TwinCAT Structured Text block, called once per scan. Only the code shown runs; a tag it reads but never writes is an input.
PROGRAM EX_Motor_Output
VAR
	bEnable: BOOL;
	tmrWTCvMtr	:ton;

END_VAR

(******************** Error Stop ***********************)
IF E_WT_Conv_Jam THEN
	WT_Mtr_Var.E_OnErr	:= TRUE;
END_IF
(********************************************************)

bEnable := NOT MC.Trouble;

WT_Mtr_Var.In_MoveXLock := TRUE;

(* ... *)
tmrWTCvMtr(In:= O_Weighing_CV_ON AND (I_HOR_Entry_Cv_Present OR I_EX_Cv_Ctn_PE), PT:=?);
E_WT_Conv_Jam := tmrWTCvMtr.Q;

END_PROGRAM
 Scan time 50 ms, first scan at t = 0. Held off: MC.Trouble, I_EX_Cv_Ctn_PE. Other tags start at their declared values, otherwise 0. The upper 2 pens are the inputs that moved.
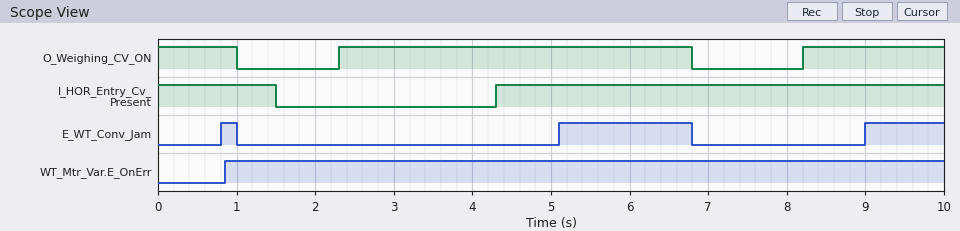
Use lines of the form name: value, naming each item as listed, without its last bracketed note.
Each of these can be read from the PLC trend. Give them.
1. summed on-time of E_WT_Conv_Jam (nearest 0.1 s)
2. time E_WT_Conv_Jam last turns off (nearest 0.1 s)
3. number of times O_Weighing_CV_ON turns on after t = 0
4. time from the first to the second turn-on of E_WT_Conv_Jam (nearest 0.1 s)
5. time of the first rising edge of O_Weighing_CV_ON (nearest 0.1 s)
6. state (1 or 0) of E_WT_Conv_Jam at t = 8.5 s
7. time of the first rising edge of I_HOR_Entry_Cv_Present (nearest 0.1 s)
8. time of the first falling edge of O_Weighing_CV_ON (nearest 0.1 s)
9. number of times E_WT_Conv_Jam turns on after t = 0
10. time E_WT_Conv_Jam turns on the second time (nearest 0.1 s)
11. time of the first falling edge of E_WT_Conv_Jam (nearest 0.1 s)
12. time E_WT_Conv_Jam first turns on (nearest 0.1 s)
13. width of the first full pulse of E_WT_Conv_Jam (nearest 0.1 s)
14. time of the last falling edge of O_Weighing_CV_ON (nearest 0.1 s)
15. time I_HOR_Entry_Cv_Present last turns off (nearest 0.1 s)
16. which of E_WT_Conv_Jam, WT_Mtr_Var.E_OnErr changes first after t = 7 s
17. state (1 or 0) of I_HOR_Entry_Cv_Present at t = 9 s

summed on-time of E_WT_Conv_Jam: 2.9 s
time E_WT_Conv_Jam last turns off: 6.8 s
number of times O_Weighing_CV_ON turns on after t = 0: 2
time from the first to the second turn-on of E_WT_Conv_Jam: 4.3 s
time of the first rising edge of O_Weighing_CV_ON: 2.3 s
state (1 or 0) of E_WT_Conv_Jam at t = 8.5 s: 0
time of the first rising edge of I_HOR_Entry_Cv_Present: 4.3 s
time of the first falling edge of O_Weighing_CV_ON: 1.0 s
number of times E_WT_Conv_Jam turns on after t = 0: 3
time E_WT_Conv_Jam turns on the second time: 5.1 s
time of the first falling edge of E_WT_Conv_Jam: 1.0 s
time E_WT_Conv_Jam first turns on: 0.8 s
width of the first full pulse of E_WT_Conv_Jam: 0.2 s
time of the last falling edge of O_Weighing_CV_ON: 6.8 s
time I_HOR_Entry_Cv_Present last turns off: 1.5 s
which of E_WT_Conv_Jam, WT_Mtr_Var.E_OnErr changes first after t = 7 s: E_WT_Conv_Jam
state (1 or 0) of I_HOR_Entry_Cv_Present at t = 9 s: 1
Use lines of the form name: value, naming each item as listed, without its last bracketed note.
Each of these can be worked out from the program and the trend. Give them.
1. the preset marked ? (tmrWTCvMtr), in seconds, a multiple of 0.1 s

the preset marked ? (tmrWTCvMtr), in seconds, a multiple of 0.1 s: 0.8 s
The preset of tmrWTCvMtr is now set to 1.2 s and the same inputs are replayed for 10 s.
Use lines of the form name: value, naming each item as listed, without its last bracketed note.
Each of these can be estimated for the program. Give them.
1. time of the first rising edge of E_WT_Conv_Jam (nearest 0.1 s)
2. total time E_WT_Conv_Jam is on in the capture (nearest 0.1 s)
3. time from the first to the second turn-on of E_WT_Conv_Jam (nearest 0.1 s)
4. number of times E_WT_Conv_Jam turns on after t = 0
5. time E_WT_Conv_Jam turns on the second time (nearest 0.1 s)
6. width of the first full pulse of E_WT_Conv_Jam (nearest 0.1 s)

time of the first rising edge of E_WT_Conv_Jam: 5.5 s
total time E_WT_Conv_Jam is on in the capture: 1.9 s
time from the first to the second turn-on of E_WT_Conv_Jam: 3.9 s
number of times E_WT_Conv_Jam turns on after t = 0: 2
time E_WT_Conv_Jam turns on the second time: 9.4 s
width of the first full pulse of E_WT_Conv_Jam: 1.3 s
